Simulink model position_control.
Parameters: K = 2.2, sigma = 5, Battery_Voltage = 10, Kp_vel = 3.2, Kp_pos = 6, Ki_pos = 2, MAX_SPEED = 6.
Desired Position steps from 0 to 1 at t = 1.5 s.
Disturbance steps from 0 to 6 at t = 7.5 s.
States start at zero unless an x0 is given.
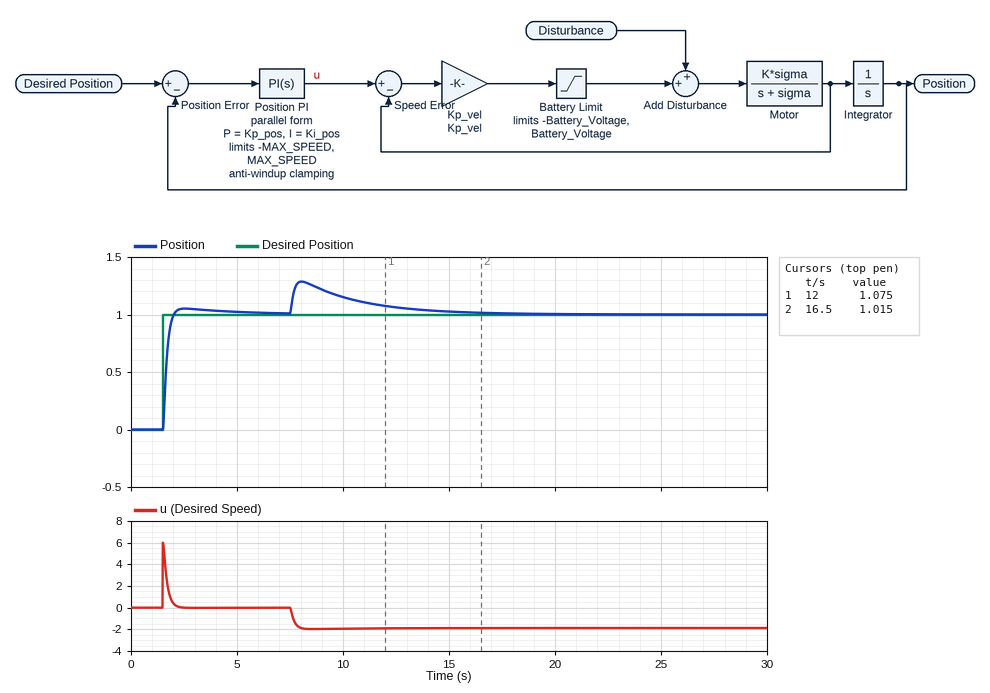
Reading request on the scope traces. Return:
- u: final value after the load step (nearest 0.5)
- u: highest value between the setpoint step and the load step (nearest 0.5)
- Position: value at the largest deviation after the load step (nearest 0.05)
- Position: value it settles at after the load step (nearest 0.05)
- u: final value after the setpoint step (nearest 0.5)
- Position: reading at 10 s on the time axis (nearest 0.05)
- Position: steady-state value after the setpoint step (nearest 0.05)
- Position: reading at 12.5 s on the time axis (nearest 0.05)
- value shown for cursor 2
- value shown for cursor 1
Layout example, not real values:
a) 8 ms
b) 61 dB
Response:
a) -2.0
b) 6.0
c) 1.30
d) 1.00
e) 0.0
f) 1.15
g) 1.00
h) 1.05
i) 1.015
j) 1.075
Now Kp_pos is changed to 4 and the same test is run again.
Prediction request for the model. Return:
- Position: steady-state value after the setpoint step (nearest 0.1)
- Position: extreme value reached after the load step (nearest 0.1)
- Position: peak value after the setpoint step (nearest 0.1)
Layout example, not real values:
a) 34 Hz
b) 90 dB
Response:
a) 1.0
b) 1.4
c) 1.1
